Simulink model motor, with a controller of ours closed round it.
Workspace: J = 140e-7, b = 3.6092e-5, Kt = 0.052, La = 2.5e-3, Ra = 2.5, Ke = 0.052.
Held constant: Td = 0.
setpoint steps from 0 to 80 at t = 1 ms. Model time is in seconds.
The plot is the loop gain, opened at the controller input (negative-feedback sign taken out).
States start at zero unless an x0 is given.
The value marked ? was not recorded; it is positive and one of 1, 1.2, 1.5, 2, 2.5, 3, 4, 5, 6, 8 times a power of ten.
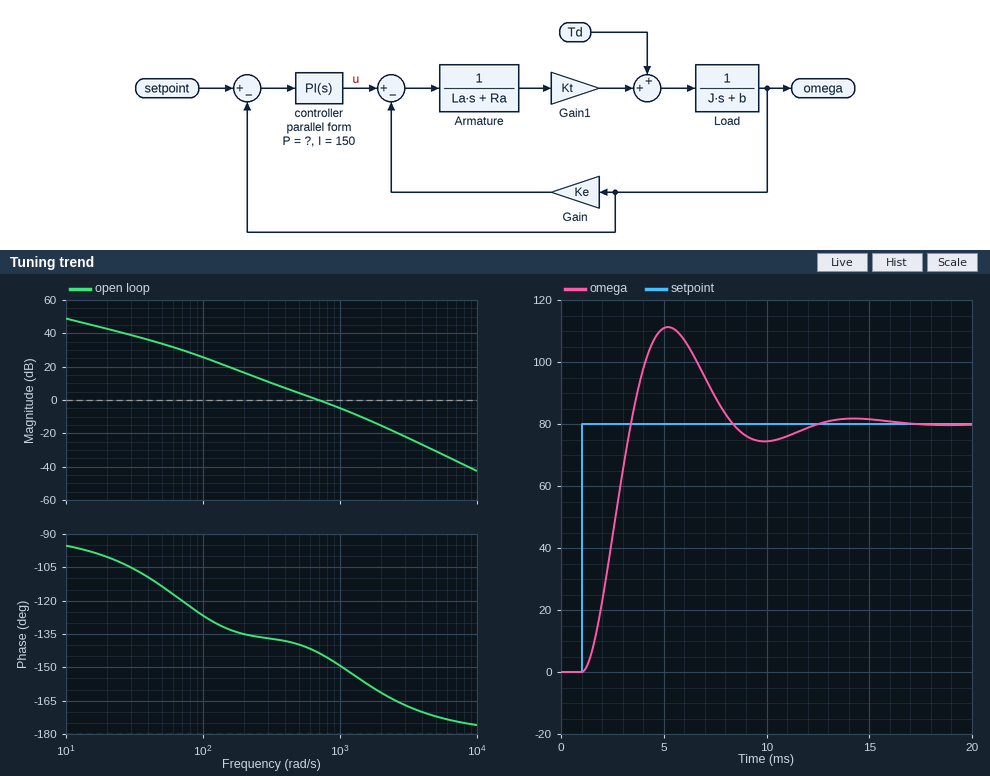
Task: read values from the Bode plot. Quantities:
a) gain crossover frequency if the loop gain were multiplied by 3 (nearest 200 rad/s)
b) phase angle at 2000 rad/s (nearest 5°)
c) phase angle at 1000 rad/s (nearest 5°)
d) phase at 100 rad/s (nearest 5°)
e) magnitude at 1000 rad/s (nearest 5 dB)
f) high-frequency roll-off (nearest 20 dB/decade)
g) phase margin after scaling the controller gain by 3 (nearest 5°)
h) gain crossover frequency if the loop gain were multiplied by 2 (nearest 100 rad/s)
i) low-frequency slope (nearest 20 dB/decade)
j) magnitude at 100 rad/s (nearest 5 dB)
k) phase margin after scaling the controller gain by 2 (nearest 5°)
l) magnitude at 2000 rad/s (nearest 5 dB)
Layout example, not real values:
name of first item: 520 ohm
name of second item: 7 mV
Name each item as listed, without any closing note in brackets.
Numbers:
gain crossover frequency if the loop gain were multiplied by 3: 1400 rad/s
phase angle at 2000 rad/s: -160°
phase angle at 1000 rad/s: -150°
phase at 100 rad/s: -125°
magnitude at 1000 rad/s: -5 dB
high-frequency roll-off: -40 dB/decade
phase margin after scaling the controller gain by 3: 25°
gain crossover frequency if the loop gain were multiplied by 2: 1100 rad/s
low-frequency slope: -20 dB/decade
magnitude at 100 rad/s: 25 dB
phase margin after scaling the controller gain by 2: 30°
magnitude at 2000 rad/s: -15 dB
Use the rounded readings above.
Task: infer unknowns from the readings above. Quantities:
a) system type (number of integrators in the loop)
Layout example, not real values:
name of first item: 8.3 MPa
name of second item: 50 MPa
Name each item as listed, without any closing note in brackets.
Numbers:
system type: 1
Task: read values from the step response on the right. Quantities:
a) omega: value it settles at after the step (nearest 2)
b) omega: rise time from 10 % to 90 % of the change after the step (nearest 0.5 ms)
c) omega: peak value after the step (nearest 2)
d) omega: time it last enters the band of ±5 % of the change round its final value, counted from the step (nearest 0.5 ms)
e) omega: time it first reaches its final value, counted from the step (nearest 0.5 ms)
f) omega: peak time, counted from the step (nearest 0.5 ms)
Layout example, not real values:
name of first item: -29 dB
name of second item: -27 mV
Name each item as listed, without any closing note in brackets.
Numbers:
omega: value it settles at after the step: 80
omega: rise time from 10 % to 90 % of the change after the step: 1.5 ms
omega: peak value after the step: 112
omega: time it last enters the band of ±5 % of the change round its final value, counted from the step: 10.0 ms
omega: time it first reaches its final value, counted from the step: 2.5 ms
omega: peak time, counted from the step: 4.0 ms
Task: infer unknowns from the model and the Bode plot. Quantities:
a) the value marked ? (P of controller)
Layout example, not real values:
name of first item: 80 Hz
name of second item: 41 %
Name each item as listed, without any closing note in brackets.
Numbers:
the value marked ?: 0.5
